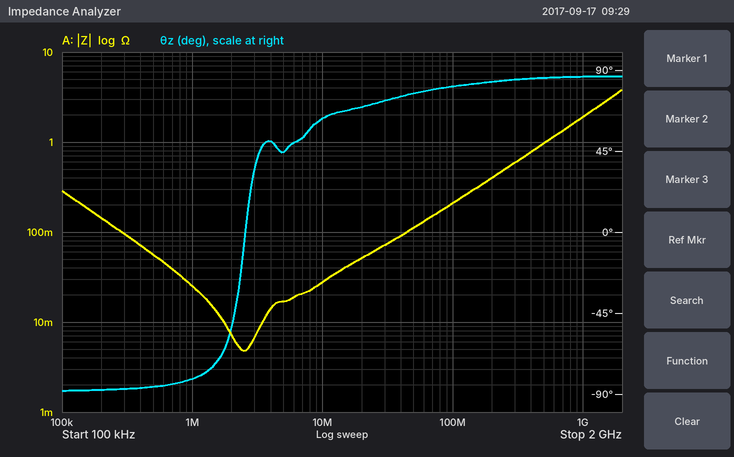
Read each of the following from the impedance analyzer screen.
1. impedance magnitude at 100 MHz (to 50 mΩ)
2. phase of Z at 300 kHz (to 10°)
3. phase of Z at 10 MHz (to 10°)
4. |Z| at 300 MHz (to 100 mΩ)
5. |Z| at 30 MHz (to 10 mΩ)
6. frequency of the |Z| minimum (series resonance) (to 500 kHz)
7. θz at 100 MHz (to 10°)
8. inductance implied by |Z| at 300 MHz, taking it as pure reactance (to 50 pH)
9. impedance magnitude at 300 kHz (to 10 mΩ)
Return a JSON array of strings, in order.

["200 mΩ", "-90°", "60°", "600 mΩ", "70 mΩ", "2.5 MHz", "80°", "300 pH", "100 mΩ"]
